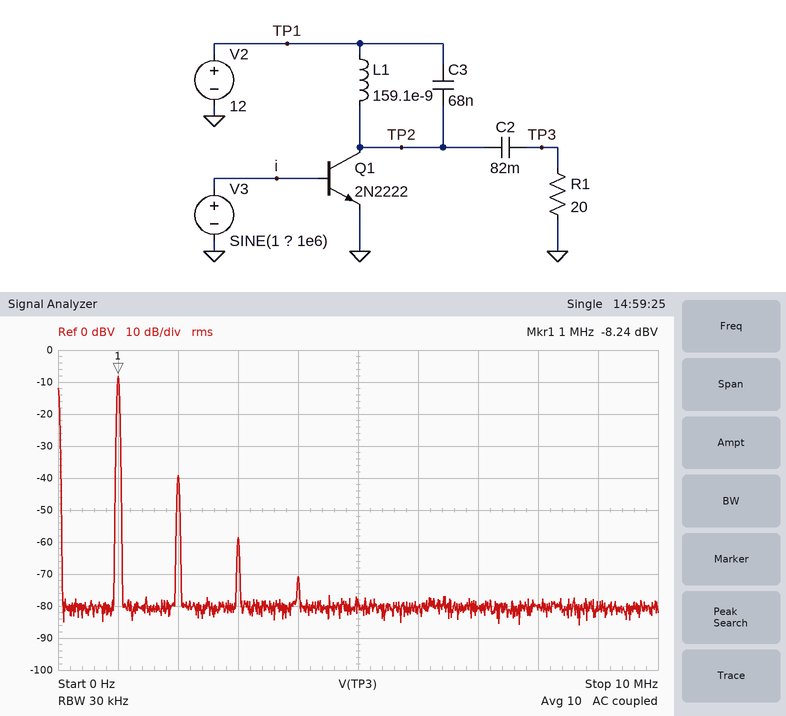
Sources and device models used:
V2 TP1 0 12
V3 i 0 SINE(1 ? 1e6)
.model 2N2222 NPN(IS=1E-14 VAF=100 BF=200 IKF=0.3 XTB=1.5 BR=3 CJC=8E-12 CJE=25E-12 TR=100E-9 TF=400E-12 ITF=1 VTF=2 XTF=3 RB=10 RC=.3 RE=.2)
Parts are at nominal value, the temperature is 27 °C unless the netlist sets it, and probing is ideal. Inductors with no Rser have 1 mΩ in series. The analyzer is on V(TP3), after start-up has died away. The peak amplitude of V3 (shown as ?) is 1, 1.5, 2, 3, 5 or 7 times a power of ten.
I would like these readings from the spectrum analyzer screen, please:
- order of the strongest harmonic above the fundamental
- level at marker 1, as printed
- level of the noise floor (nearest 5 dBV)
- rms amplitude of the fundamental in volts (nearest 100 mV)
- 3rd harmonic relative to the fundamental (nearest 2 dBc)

2
-8.24 dBV
-80 dBV
400 mV
-50 dBc
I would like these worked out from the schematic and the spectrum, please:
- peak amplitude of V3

150 mV
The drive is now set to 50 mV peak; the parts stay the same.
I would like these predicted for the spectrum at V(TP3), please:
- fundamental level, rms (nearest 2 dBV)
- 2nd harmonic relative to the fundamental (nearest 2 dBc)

-18 dBV
-38 dBc
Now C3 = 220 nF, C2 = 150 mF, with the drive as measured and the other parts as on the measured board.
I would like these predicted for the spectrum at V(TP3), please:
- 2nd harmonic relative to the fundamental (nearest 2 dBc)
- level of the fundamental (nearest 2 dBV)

-50 dBc
-4 dBV
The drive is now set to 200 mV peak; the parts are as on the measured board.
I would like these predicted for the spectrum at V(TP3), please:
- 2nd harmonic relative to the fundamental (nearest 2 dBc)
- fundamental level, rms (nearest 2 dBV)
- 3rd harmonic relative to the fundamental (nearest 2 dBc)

-32 dBc
-6 dBV
-42 dBc
